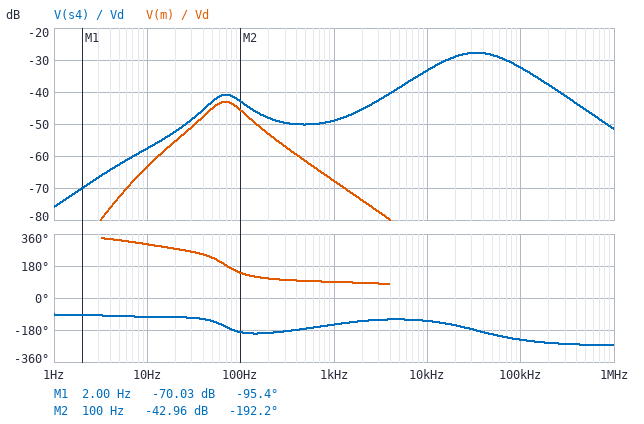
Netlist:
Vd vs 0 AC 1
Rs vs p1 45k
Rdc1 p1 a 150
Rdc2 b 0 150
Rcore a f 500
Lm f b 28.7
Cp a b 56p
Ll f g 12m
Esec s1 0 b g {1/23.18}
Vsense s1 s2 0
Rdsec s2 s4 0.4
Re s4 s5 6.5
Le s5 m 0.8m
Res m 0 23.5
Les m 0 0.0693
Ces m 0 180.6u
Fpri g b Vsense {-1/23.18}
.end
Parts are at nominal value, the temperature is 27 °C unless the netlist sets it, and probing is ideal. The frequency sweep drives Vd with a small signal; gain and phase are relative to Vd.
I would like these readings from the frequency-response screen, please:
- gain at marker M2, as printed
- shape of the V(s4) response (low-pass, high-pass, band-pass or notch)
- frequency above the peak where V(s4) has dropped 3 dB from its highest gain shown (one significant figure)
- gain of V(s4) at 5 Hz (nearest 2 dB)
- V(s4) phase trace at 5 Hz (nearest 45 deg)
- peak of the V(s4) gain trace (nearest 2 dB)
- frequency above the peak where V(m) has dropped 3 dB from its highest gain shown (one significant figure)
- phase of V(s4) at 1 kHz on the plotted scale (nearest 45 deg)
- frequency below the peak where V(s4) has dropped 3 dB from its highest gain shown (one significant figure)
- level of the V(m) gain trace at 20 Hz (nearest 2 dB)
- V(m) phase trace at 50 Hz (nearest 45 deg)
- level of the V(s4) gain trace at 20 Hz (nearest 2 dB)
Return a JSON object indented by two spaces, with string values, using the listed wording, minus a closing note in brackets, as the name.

{
  "gain at marker M2, as printed": "-42.96 dB",
  "shape of the V(s4) response": "band-pass",
  "frequency above the peak where V(s4) has dropped 3 dB from its highest gain shown": "80 kHz",
  "gain of V(s4) at 5 Hz": "-62 dB",
  "V(s4) phase trace at 5 Hz": "-90 deg",
  "peak of the V(s4) gain trace": "-28 dB",
  "frequency above the peak where V(m) has dropped 3 dB from its highest gain shown": "100 Hz",
  "phase of V(s4) at 1 kHz on the plotted scale": "-135 deg",
  "frequency below the peak where V(s4) has dropped 3 dB from its highest gain shown": "10 kHz",
  "level of the V(m) gain trace at 20 Hz": "-56 dB",
  "V(m) phase trace at 50 Hz": "225 deg",
  "level of the V(s4) gain trace at 20 Hz": "-52 dB"
}
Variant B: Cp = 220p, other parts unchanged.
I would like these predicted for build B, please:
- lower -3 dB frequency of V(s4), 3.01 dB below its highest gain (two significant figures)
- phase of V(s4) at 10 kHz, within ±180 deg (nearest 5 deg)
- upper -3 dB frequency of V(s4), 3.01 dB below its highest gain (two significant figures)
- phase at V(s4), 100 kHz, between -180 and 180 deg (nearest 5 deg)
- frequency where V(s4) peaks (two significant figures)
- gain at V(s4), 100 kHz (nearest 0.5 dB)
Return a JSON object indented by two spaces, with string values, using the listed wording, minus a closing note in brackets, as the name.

{
  "lower -3 dB frequency of V(s4), 3.01 dB below its highest gain": "10 kHz",
  "phase of V(s4) at 10 kHz, within ±180 deg": "-140 deg",
  "upper -3 dB frequency of V(s4), 3.01 dB below its highest gain": "28 kHz",
  "phase at V(s4), 100 kHz, between -180 and 180 deg": "100 deg",
  "frequency where V(s4) peaks": "17 kHz",
  "gain at V(s4), 100 kHz": "-43.5 dB"
}
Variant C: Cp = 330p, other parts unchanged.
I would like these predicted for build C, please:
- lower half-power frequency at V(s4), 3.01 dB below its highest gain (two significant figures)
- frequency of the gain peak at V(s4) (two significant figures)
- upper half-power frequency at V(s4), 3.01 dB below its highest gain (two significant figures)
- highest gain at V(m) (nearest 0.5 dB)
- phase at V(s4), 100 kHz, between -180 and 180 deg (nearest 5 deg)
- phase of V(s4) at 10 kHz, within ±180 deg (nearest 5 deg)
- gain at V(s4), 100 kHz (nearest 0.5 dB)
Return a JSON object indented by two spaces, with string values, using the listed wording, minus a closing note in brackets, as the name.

{
  "lower half-power frequency at V(s4), 3.01 dB below its highest gain": "9.0 kHz",
  "frequency of the gain peak at V(s4)": "14 kHz",
  "upper half-power frequency at V(s4), 3.01 dB below its highest gain": "21 kHz",
  "highest gain at V(m)": "-43.0 dB",
  "phase at V(s4), 100 kHz, between -180 and 180 deg": "95 deg",
  "phase of V(s4) at 10 kHz, within ±180 deg": "-150 deg",
  "gain at V(s4), 100 kHz": "-47.0 dB"
}
